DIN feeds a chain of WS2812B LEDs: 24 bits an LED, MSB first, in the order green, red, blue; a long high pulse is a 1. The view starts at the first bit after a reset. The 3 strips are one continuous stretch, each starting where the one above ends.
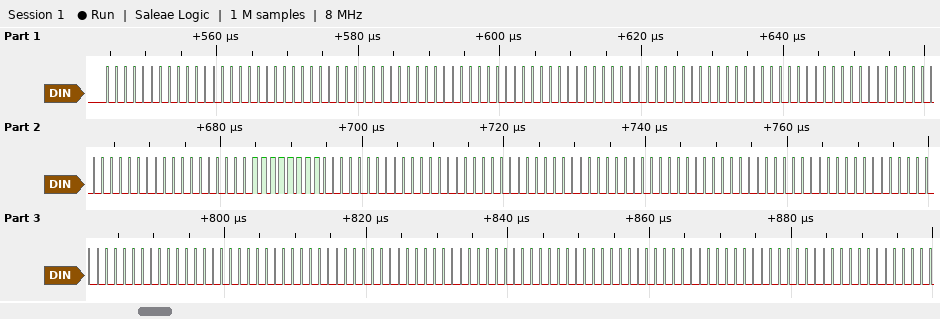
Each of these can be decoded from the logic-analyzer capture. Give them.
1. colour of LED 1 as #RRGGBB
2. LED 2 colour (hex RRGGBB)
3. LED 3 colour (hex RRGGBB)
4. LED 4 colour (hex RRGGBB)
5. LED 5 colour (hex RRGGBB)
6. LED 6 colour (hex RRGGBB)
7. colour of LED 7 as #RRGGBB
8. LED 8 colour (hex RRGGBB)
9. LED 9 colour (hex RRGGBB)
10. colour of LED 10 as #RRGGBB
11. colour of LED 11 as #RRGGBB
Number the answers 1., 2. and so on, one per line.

1. #000000
2. #000000
3. #000000
4. #000000
5. #0000FF
6. #000000
7. #000000
8. #000000
9. #000000
10. #000000
11. #000000
